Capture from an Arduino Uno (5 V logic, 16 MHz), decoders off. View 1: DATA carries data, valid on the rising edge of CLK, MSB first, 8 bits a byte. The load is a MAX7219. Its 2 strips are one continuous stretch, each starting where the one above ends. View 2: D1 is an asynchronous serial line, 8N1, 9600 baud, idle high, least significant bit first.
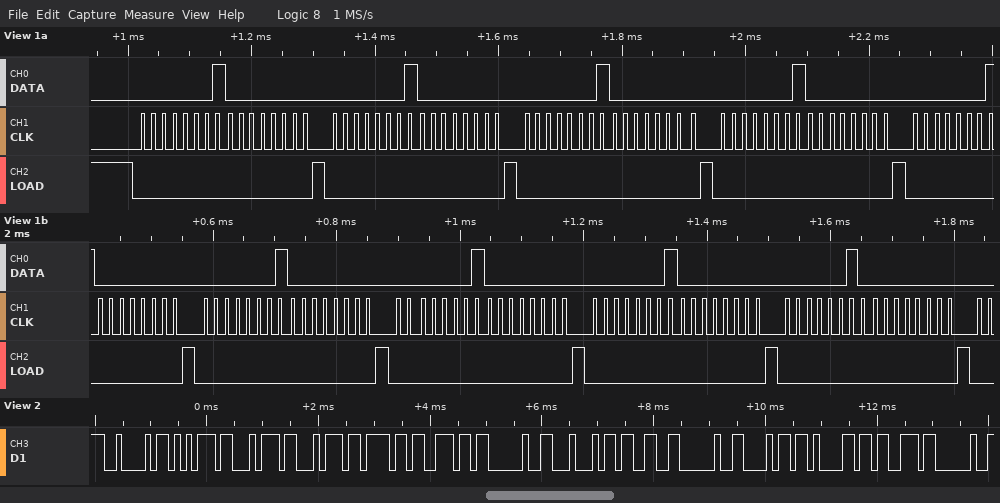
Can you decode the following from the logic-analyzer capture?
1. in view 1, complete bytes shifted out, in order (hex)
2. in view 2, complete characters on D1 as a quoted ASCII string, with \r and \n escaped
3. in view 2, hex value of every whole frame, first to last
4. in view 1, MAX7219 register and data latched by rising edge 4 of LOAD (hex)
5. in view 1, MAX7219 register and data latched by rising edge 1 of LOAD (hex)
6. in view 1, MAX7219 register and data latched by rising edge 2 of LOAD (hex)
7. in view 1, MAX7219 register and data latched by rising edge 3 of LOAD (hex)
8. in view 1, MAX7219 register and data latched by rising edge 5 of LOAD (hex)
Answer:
01 00 01 00 01 00 01 00 01 00 01 00 01 00 01 00 02 00
"Button D3 has "
42 75 74 74 6F 6E 20 44 33 20 68 61 73 20
register 0x1, data 0x00
register 0x1, data 0x00
register 0x1, data 0x00
register 0x1, data 0x00
register 0x1, data 0x00
